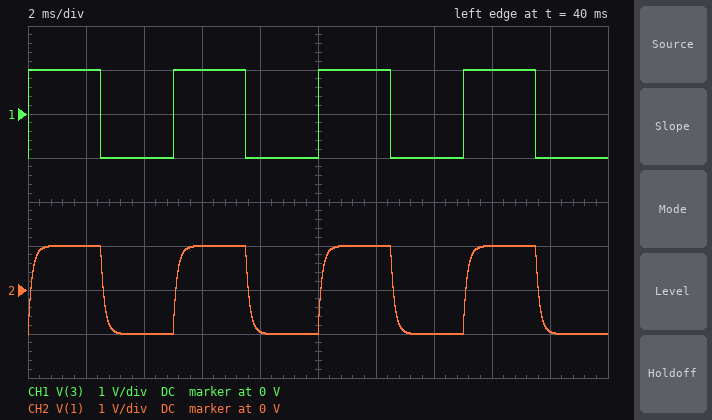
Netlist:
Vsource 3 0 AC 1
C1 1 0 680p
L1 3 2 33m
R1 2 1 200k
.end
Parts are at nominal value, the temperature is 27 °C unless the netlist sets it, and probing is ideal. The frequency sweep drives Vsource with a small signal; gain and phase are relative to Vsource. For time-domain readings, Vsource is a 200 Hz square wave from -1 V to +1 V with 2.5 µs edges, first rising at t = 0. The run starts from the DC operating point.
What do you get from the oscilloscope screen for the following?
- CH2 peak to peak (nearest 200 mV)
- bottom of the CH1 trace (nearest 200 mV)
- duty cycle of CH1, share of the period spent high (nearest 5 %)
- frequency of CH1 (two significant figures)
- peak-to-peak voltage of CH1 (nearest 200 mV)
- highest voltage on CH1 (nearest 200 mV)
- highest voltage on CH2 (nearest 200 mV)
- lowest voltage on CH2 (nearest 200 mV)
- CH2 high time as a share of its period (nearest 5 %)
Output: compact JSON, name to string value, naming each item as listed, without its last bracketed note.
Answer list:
{"CH2 peak to peak": "2.0 V", "bottom of the CH1 trace": "-1.0 V", "duty cycle of CH1, share of the period spent high": "50 %", "frequency of CH1": "200 Hz", "peak-to-peak voltage of CH1": "2.0 V", "highest voltage on CH1": "1.0 V", "highest voltage on CH2": "1.0 V", "lowest voltage on CH2": "-1.0 V", "CH2 high time as a share of its period": "50 %"}
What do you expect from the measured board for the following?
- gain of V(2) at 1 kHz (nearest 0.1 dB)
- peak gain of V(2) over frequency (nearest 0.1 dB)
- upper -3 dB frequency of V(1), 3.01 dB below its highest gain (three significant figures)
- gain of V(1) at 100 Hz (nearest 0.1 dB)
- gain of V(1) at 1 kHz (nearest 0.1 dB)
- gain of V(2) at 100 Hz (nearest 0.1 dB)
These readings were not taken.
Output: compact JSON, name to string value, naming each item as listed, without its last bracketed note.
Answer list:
{"gain of V(2) at 1 kHz": "0 dB", "peak gain of V(2) over frequency": "0 dB", "upper -3 dB frequency of V(1), 3.01 dB below its highest gain": "1.17 kHz", "gain of V(1) at 100 Hz": "0 dB", "gain of V(1) at 1 kHz": "-2.4 dB", "gain of V(2) at 100 Hz": "0 dB"}
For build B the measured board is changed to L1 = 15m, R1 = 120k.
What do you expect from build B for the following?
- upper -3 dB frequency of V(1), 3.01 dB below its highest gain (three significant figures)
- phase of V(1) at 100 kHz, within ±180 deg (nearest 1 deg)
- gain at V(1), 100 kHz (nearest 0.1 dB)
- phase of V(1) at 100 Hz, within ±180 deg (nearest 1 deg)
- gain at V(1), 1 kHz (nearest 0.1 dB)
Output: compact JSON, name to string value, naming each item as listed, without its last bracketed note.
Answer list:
{"upper -3 dB frequency of V(1), 3.01 dB below its highest gain": "1.95 kHz", "phase of V(1) at 100 kHz, within ±180 deg": "-93 deg", "gain at V(1), 100 kHz": "-34.2 dB", "phase of V(1) at 100 Hz, within ±180 deg": "-3 deg", "gain at V(1), 1 kHz": "-1.0 dB"}
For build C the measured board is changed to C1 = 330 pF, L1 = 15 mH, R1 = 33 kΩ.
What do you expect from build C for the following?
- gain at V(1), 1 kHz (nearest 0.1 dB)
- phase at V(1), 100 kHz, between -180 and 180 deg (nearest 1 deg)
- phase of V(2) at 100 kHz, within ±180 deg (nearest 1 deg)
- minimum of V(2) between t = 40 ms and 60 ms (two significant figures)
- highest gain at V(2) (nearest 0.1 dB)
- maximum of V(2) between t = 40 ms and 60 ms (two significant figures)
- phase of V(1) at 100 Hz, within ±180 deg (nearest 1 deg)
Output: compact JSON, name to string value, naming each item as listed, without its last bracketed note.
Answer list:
{"gain at V(1), 1 kHz": "0 dB", "phase at V(1), 100 kHz, between -180 and 180 deg": "-98 deg", "phase of V(2) at 100 kHz, within ±180 deg": "-16 deg", "minimum of V(2) between t = 40 ms and 60 ms": "-1.1 V", "highest gain at V(2)": "0.3 dB", "maximum of V(2) between t = 40 ms and 60 ms": "1.1 V", "phase of V(1) at 100 Hz, within ±180 deg": "0 deg"}
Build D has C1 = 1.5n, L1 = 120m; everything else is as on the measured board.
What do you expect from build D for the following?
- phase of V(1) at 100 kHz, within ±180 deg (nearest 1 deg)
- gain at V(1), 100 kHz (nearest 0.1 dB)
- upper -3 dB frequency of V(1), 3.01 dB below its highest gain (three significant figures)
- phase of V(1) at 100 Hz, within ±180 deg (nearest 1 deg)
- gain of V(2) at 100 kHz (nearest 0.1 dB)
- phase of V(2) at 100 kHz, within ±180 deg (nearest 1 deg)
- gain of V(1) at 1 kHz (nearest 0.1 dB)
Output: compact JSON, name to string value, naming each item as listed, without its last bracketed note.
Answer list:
{"phase of V(1) at 100 kHz, within ±180 deg": "-110 deg", "gain at V(1), 100 kHz": "-46.1 dB", "upper -3 dB frequency of V(1), 3.01 dB below its highest gain": "532 Hz", "phase of V(1) at 100 Hz, within ±180 deg": "-11 deg", "gain of V(2) at 100 kHz": "-0.6 dB", "phase of V(2) at 100 kHz, within ±180 deg": "-21 deg", "gain of V(1) at 1 kHz": "-6.6 dB"}
